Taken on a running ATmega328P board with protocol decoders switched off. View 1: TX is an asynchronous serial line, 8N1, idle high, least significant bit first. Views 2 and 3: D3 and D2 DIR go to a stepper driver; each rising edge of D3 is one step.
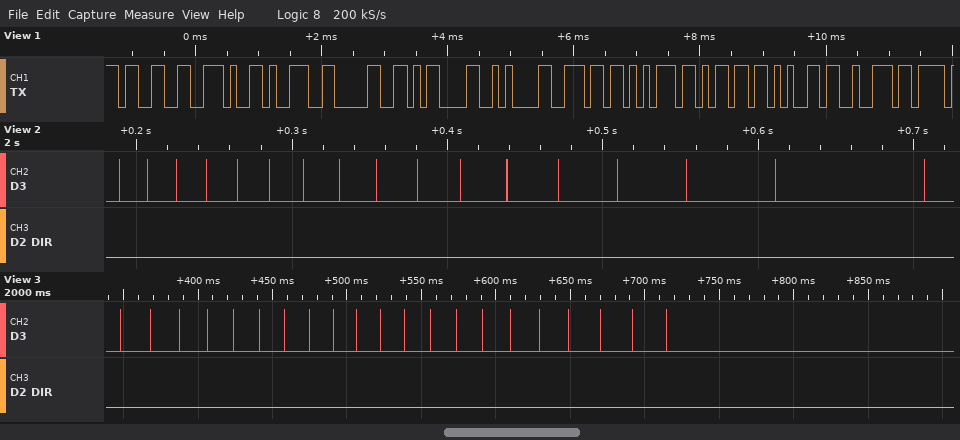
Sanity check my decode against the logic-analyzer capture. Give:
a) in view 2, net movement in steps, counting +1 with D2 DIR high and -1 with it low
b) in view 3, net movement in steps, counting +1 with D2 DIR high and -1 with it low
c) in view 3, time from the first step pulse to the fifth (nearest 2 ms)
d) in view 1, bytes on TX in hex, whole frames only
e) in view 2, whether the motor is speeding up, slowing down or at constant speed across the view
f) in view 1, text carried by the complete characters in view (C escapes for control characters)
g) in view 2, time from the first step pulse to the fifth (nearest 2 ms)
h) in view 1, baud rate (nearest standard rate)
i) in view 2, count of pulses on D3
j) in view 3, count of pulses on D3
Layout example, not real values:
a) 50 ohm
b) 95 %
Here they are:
a) -17
b) -21
c) 76 ms
d) 33 2E 39 30 0D 0A 6E 75 6D 65 72
e) slowing down
f) "3.90\r\nnumer"
g) 76 ms
h) 9600 baud
i) 17
j) 21
